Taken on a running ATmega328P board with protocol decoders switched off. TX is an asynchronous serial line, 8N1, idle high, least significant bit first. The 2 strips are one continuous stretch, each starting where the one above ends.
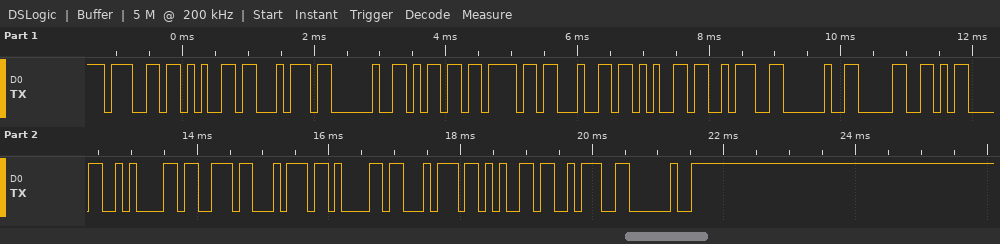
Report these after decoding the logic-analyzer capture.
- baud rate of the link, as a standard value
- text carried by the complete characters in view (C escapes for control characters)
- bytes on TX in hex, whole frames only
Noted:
9600 baud
"get mode: 0\r\nstate: "
67 65 74 20 6D 6F 64 65 3A 20 30 0D 0A 73 74 61 74 65 3A 20
